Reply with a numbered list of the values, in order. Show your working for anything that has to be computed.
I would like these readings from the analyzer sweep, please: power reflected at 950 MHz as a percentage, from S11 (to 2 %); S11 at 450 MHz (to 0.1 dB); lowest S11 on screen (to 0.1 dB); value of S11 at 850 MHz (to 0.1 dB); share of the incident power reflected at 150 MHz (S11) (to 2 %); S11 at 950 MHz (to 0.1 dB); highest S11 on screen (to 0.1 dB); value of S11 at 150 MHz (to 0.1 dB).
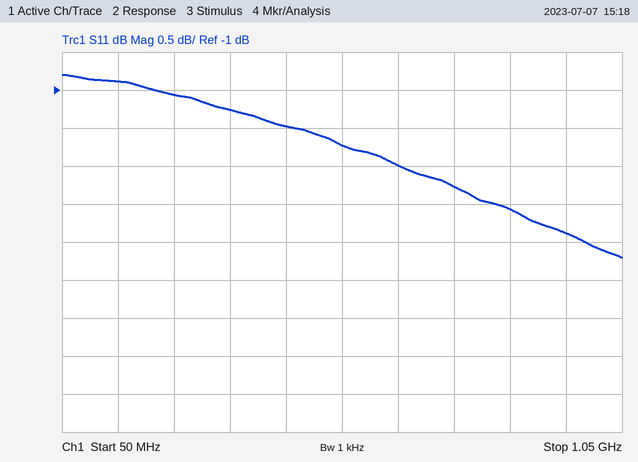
1. 10^(-2.9/10) ≈ 51.3 %, so 52 % to the nearest 2 %
2. -1.5 dB
3. -3.2 dB
4. -2.6 dB
5. 10^(-0.9/10) ≈ 81.3 %, so 82 % to the nearest 2 %
6. -2.9 dB
7. -0.8 dB
8. -0.9 dB
